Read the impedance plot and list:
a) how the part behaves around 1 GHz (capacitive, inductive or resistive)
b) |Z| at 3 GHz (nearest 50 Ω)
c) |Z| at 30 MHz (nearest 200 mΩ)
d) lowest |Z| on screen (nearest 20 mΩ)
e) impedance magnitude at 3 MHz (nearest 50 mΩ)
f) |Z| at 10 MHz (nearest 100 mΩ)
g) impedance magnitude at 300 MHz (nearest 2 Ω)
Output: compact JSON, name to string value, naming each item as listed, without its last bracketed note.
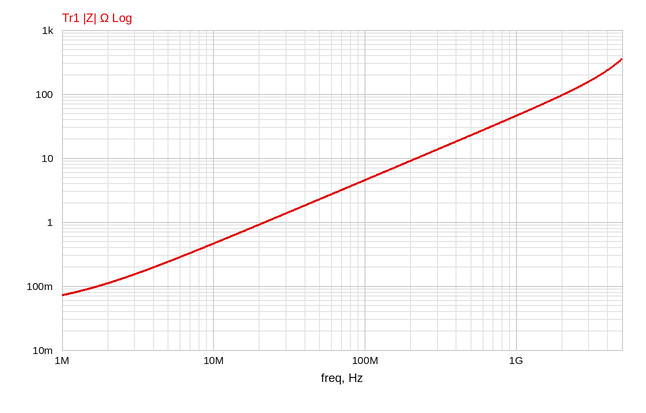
{"how the part behaves around 1 GHz": "inductive", "|Z| at 3 GHz": "150 Ω", "|Z| at 30 MHz": "1.4 Ω", "lowest |Z| on screen": "80 mΩ", "impedance magnitude at 3 MHz": "150 mΩ", "|Z| at 10 MHz": "500 mΩ", "impedance magnitude at 300 MHz": "14 Ω"}
